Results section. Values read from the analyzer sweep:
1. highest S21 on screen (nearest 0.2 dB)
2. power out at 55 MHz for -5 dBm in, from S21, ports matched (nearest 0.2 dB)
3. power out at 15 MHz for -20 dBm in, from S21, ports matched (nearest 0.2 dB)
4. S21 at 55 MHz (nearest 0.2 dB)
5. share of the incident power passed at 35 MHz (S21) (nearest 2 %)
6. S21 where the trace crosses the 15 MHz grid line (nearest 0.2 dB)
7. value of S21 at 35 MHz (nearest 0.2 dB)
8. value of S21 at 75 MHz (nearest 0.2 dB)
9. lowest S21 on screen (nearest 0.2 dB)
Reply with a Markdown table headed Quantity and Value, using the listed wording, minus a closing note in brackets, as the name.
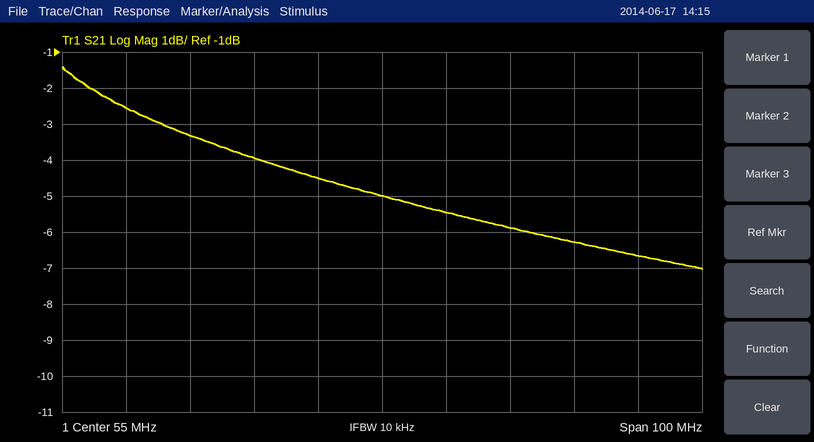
| Quantity | Value |
|---|---|
| highest S21 on screen | -1.4 dB |
| power out at 55 MHz for -5 dBm in, from S21, ports matched | -10.0 dBm |
| power out at 15 MHz for -20 dBm in, from S21, ports matched | -22.6 dBm |
| S21 at 55 MHz | -5.0 dB |
| share of the incident power passed at 35 MHz (S21) | 40 % |
| S21 where the trace crosses the 15 MHz grid line | -2.6 dB |
| value of S21 at 35 MHz | -4.0 dB |
| value of S21 at 75 MHz | -5.8 dB |
| lowest S21 on screen | -7.0 dB |
